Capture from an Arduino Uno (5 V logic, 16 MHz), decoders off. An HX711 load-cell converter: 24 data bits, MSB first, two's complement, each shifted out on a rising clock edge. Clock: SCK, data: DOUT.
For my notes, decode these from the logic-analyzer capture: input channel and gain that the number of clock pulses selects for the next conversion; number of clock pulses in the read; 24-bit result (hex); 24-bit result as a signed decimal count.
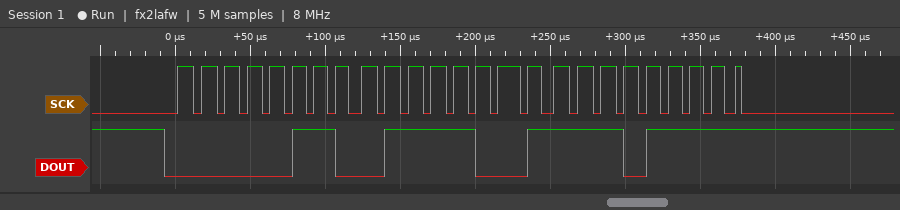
channel A, gain 128
25
0x0679EF
424431
